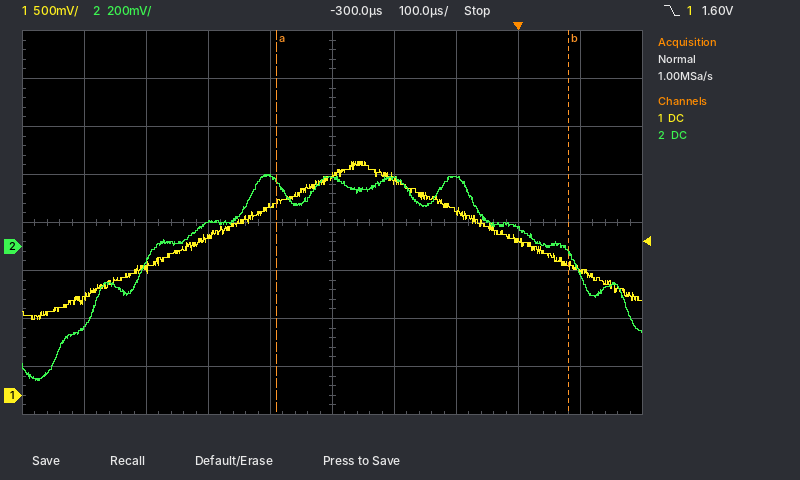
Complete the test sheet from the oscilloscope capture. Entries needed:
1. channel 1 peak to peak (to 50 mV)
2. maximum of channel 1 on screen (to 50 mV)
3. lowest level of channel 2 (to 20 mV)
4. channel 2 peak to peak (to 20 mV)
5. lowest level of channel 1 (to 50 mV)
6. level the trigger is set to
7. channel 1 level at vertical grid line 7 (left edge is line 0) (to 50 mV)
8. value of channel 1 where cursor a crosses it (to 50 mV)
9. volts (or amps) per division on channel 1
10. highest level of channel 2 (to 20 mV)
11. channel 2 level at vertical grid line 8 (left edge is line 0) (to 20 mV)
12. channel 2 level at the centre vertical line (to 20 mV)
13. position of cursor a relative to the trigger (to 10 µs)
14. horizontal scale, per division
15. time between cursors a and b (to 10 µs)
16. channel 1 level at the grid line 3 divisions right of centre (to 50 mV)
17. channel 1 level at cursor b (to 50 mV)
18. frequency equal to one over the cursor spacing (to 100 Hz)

1.65 V
2.45 V
-560 mV
860 mV
800 mV
1.60 V
1.90 V
2.00 V
500 mV
300 mV
80 mV
280 mV
-390 µs
100 µs
470 µs
1.60 V
1.35 V
2.1 kHz
